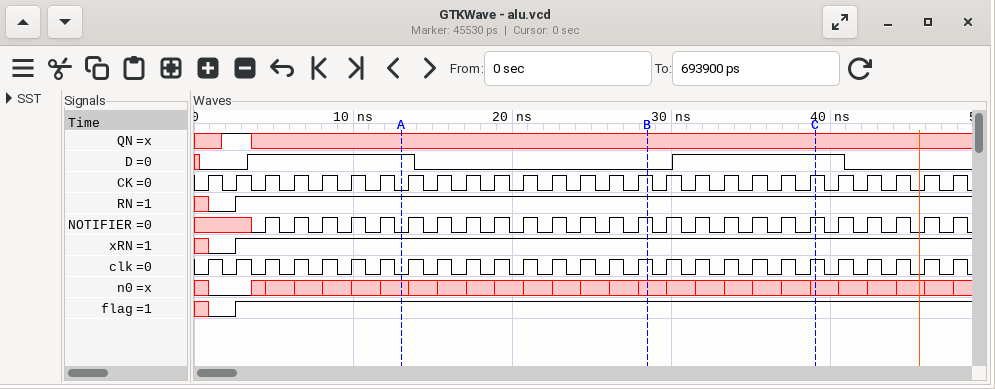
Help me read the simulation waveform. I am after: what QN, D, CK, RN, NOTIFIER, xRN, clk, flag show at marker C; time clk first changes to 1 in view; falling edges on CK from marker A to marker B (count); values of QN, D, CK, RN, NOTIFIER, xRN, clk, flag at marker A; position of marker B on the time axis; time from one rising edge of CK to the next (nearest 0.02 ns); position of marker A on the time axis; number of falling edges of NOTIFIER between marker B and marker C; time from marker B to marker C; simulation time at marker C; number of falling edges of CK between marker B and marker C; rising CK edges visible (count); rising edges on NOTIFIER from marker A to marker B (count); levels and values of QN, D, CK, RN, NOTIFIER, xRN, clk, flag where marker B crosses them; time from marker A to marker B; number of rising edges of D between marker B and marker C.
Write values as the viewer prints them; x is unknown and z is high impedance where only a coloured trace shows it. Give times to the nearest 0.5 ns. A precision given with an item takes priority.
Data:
QN=x, D=1, CK=1, RN=1, NOTIFIER=1, xRN=1, clk=1, flag=1
1 ns
8
QN=x, D=1, CK=0, RN=1, NOTIFIER=0, xRN=1, clk=0, flag=1
28.5 ns
1.8 ns
13 ns
6
10.5 ns
39 ns
6
27
9
QN=x, D=0, CK=1, RN=1, NOTIFIER=1, xRN=1, clk=1, flag=1
15.5 ns
1
